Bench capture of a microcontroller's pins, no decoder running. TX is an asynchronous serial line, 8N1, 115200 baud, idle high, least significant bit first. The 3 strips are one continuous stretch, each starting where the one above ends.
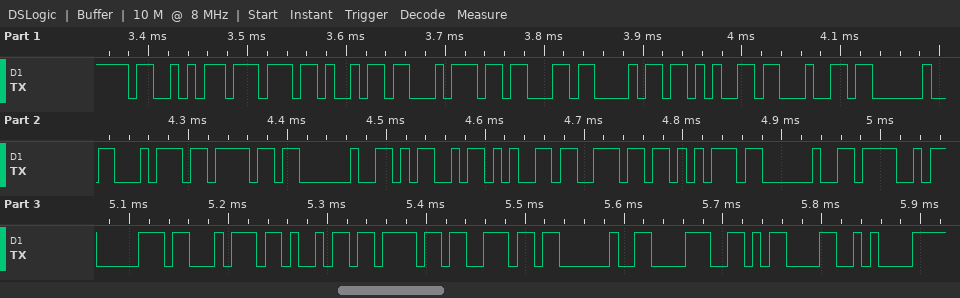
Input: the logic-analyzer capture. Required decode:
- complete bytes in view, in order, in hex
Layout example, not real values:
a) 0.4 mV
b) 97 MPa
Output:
a) 53 77 69 74 63 68 65 64 20 74 6F 20 4D 65 6E 75 20 4F 70 74 69 6F 6E 20 38 0D 0A
